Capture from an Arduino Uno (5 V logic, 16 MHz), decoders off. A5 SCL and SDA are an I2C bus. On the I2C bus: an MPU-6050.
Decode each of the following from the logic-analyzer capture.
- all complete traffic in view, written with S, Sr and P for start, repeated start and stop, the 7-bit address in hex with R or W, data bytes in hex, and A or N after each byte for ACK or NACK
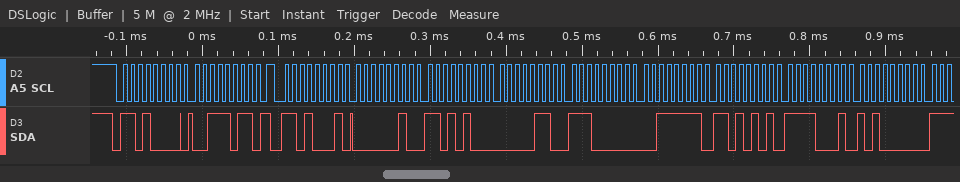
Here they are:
S 68W A 3B A Sr 68R A 02 A D4 A 06 A E0 A 3F A D5 A F1 A A0 A
